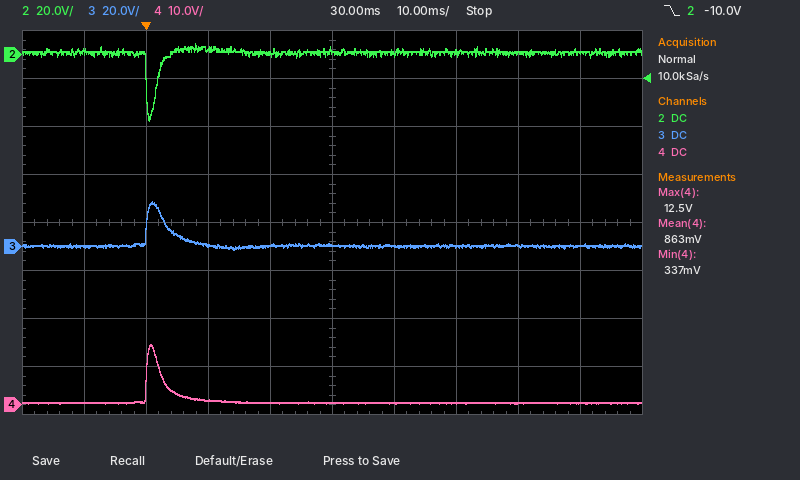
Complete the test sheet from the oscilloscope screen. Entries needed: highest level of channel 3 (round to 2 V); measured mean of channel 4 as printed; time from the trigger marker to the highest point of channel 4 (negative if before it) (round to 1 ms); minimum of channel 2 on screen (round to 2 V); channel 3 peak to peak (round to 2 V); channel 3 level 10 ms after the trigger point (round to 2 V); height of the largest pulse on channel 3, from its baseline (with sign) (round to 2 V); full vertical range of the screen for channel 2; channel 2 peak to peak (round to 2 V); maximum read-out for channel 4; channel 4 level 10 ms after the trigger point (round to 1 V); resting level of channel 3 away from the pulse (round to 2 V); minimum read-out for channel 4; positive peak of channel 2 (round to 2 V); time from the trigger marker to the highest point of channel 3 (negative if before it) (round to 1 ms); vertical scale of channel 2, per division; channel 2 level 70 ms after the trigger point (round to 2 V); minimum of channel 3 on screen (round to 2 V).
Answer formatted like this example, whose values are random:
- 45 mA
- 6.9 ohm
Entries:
- 18 V
- 863 mV
- +1 ms
- -28 V
- 20 V
- 0 V
- +18 V
- 160 V
- 32 V
- 12.5 V
- 1 V
- 0 V
- 337 mV
- 4 V
- +1 ms
- 20 V
- 0 V
- -2 V
